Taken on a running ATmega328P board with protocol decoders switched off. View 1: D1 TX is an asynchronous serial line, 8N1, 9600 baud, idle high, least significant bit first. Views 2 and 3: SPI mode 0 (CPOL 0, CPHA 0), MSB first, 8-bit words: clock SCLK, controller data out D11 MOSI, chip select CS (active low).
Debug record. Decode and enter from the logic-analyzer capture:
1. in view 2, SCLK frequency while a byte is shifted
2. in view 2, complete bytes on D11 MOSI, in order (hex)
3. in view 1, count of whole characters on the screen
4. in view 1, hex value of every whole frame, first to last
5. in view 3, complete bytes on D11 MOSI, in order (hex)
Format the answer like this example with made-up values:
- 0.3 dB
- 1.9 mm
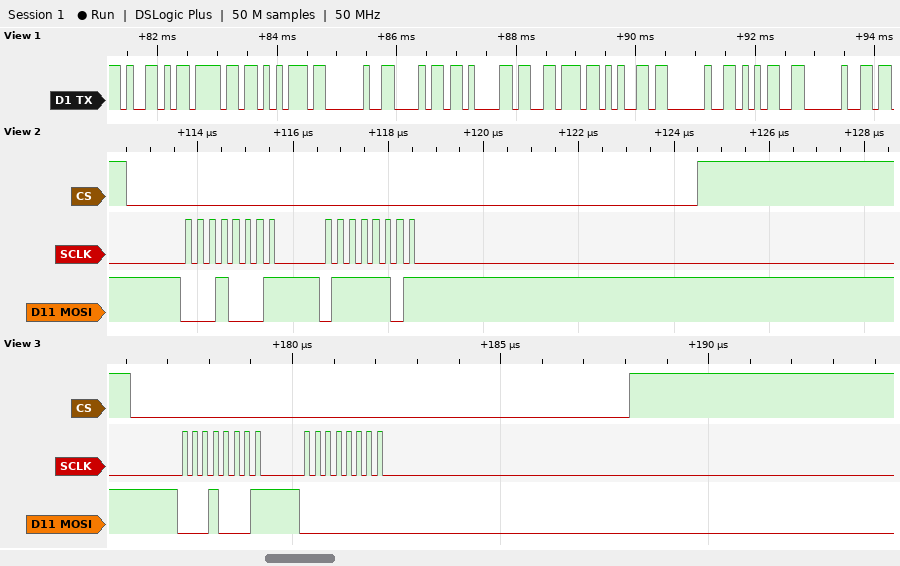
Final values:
- 4 MHz
- 0x11 0x7D
- 11
- 59 6F 75 20 68 61 76 65 20 35 20
- 11 00
